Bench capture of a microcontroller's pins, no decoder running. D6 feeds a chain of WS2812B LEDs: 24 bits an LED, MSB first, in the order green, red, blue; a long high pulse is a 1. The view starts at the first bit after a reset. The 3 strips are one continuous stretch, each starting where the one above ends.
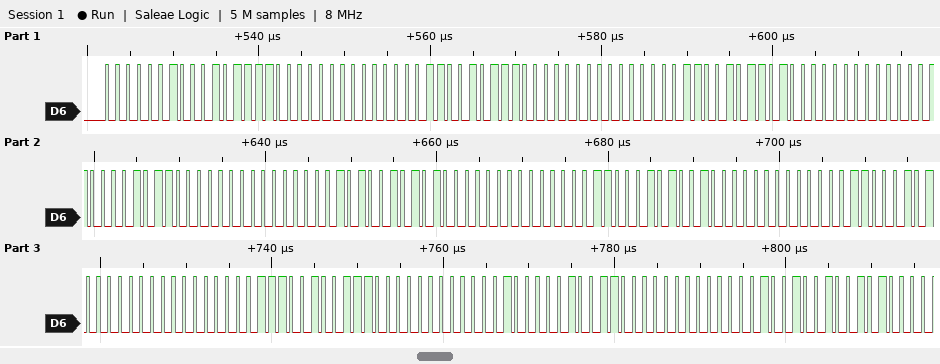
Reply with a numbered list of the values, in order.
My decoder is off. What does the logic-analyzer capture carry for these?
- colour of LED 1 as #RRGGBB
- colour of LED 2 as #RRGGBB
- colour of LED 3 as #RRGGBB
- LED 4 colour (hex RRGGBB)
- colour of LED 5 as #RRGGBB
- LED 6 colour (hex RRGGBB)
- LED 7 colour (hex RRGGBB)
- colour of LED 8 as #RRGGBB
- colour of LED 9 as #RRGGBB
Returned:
1. #2F0200
2. #2E0300
3. #2D0300
4. #2C0400
5. #2A0500
6. #290600
7. #280600
8. #270700
9. #260800
